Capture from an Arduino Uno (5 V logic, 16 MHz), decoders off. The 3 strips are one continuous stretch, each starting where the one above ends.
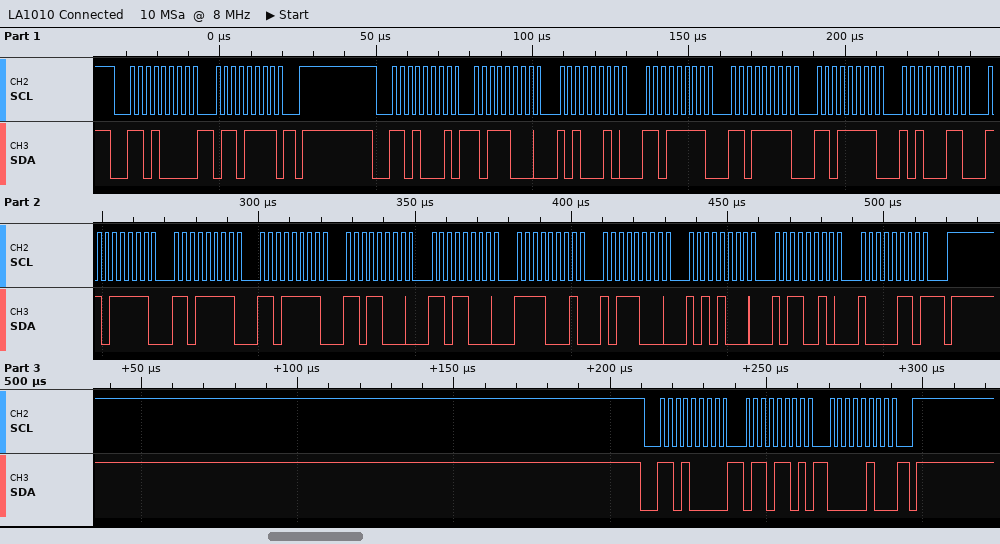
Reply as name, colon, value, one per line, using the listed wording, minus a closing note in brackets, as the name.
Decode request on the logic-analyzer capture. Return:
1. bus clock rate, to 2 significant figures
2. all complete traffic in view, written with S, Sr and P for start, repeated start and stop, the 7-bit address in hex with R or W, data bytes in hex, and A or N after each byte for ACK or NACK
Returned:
bus clock rate, to 2 significant figures: 400 kHz
all complete traffic in view, written with S, Sr and P for start, repeated start and stop, the 7-bit address in hex with R or W, data bytes in hex, and A or N after each byte for ACK or NACK: S 68W A 6F A P S 68R A B8 A A2 A DF A DF A DF A A3 A DF A DF A DF A D8 A D8 A F1 A B8 A A8 A B2 A 86 N P S 68W A 6D A 04 A P
